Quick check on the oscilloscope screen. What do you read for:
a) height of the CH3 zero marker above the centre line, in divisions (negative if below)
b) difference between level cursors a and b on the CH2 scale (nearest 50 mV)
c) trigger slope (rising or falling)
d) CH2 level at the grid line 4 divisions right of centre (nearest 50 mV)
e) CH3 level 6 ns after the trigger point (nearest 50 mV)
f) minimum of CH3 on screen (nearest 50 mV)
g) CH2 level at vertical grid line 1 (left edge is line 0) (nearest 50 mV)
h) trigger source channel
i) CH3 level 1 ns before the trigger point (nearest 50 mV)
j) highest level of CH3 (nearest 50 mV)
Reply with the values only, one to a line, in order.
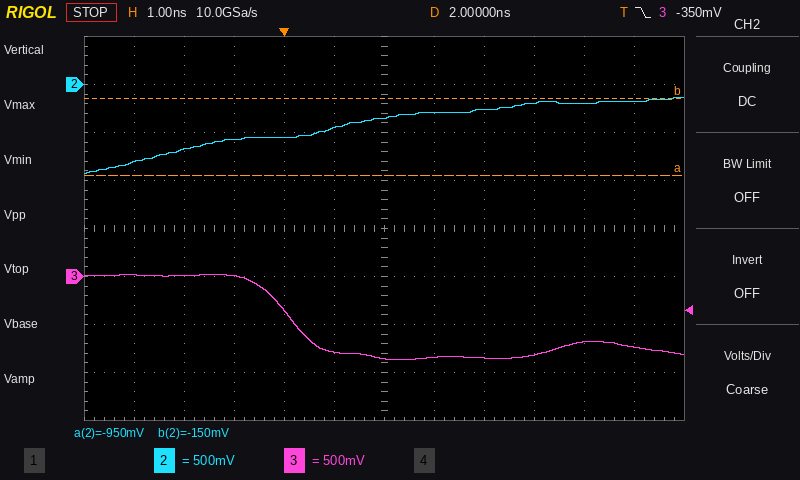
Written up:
-1.0 div
800 mV
falling
-200 mV
-700 mV
-850 mV
-800 mV
CH3
0 mV
0 mV
